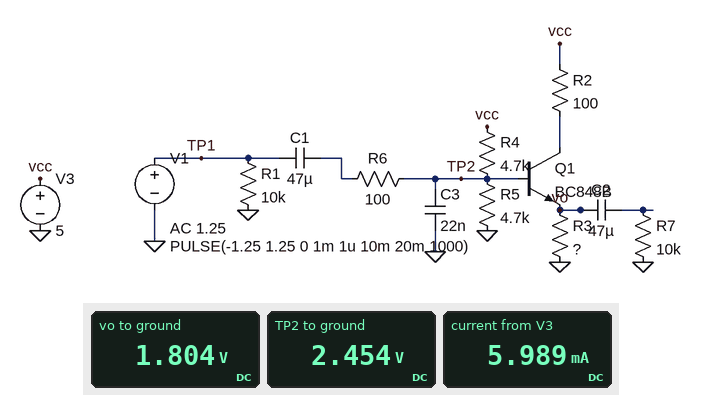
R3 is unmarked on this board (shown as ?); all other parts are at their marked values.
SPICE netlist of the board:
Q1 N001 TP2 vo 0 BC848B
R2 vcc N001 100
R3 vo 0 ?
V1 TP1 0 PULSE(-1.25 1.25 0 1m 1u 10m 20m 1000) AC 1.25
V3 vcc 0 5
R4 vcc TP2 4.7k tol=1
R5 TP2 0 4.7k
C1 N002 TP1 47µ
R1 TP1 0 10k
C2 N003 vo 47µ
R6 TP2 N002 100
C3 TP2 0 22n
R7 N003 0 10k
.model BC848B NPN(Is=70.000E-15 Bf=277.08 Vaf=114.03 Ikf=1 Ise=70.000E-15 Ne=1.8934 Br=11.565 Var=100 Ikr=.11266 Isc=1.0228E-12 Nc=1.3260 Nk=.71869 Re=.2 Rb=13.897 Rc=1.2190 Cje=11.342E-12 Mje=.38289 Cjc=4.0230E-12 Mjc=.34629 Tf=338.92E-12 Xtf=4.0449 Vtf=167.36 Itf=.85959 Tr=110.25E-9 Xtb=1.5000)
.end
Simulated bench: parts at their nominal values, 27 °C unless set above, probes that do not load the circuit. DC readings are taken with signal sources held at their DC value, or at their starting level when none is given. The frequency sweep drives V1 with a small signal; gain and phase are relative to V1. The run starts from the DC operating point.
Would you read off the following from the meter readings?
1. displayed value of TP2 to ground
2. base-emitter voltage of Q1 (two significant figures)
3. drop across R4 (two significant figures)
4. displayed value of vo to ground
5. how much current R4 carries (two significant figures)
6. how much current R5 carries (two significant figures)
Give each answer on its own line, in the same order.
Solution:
2.454 V
650 mV
2.5 V
1.804 V
540 µA
520 µA
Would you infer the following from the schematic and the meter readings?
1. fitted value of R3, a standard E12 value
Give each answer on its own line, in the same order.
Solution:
330 Ω
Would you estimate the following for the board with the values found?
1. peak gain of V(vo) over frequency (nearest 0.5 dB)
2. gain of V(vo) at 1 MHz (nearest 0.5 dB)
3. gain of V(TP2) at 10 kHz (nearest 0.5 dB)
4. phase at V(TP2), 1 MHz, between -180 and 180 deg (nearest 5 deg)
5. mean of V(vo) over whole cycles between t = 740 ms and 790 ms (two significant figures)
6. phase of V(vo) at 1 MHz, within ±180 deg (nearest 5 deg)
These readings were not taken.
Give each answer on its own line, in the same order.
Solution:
-0.5 dB
-23.0 dB
-0.5 dB
-85 deg
1.8 V
-85 deg
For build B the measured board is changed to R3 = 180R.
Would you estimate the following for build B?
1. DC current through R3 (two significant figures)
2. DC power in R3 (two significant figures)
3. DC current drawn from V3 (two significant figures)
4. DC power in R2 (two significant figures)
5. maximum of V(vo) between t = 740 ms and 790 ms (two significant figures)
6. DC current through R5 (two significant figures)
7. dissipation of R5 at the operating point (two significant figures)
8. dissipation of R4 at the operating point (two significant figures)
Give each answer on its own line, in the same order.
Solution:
9.7 mA
17 mW
10 mA
9.4 mW
2.9 V
510 µA
1.2 mW
1.4 mW
